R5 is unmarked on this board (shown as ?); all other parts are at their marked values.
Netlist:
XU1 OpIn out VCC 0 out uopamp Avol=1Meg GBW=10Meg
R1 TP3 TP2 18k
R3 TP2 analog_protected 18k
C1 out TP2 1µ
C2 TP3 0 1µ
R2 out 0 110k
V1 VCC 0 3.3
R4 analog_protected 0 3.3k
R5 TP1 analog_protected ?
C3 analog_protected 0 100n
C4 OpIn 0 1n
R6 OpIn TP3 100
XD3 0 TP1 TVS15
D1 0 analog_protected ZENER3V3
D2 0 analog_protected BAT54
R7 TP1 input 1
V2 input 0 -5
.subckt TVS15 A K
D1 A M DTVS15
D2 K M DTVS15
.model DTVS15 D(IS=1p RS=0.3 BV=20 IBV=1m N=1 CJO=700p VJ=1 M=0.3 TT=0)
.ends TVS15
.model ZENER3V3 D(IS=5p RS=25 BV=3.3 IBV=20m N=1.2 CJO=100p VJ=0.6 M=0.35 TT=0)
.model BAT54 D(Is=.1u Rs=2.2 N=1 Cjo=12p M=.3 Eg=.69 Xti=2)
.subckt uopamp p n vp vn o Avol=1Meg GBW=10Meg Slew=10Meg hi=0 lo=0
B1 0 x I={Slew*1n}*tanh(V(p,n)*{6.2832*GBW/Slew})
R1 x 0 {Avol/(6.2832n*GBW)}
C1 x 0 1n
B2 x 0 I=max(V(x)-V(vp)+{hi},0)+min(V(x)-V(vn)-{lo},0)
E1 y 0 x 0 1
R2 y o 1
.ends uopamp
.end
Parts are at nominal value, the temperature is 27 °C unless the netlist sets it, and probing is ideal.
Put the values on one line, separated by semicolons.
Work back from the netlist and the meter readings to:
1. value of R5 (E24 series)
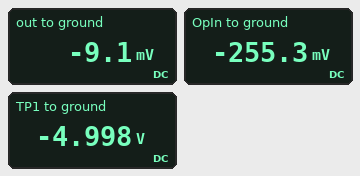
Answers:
2.7 kΩ
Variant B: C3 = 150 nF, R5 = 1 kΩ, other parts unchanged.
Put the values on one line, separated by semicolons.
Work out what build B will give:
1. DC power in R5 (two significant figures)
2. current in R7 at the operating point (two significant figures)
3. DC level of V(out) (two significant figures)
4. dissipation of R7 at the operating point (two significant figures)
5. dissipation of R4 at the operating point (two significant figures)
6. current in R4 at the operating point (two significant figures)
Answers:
22 mW; 4.7 mA; -9.4 mV; 22 µW; 25 µW; 87 µA
